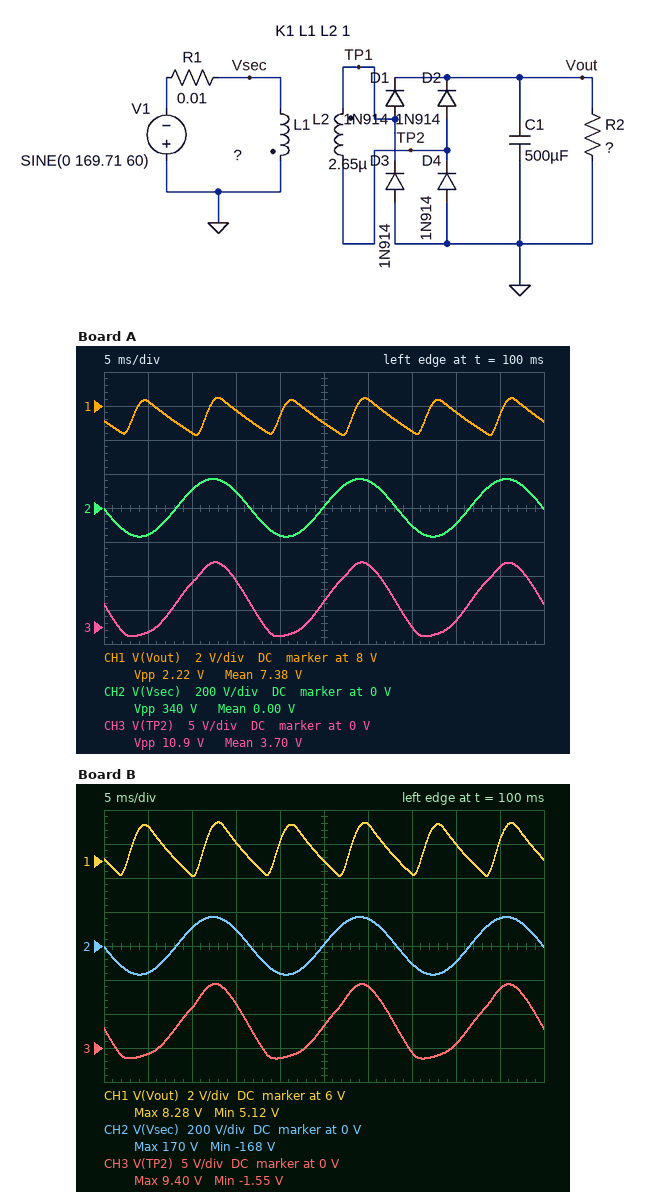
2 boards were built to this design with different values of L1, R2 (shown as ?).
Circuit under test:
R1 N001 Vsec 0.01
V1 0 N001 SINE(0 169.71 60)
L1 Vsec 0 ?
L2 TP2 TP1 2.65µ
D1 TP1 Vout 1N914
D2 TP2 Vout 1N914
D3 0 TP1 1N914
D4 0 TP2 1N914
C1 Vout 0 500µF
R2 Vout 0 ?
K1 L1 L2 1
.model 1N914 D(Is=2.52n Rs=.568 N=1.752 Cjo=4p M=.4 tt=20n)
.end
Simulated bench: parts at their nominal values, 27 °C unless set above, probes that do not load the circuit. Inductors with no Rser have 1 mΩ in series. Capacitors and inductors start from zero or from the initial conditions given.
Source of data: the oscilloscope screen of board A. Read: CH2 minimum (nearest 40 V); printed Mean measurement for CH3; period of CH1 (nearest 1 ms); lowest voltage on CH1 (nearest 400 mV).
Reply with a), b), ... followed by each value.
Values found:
a) -160 V
b) 3.70 V
c) 8 ms
d) 6.4 V
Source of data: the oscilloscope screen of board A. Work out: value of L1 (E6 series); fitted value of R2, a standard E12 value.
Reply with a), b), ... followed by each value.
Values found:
a) 680 µH
b) 39 Ω
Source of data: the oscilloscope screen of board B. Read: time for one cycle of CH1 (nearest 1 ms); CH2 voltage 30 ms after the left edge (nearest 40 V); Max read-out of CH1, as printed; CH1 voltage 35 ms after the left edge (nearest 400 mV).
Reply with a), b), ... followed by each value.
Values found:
a) 8 ms
b) 160 V
c) 8.28 V
d) 5.2 V
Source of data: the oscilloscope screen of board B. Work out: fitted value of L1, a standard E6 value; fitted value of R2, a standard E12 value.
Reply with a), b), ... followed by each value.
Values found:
a) 680 µH
b) 22 Ω
